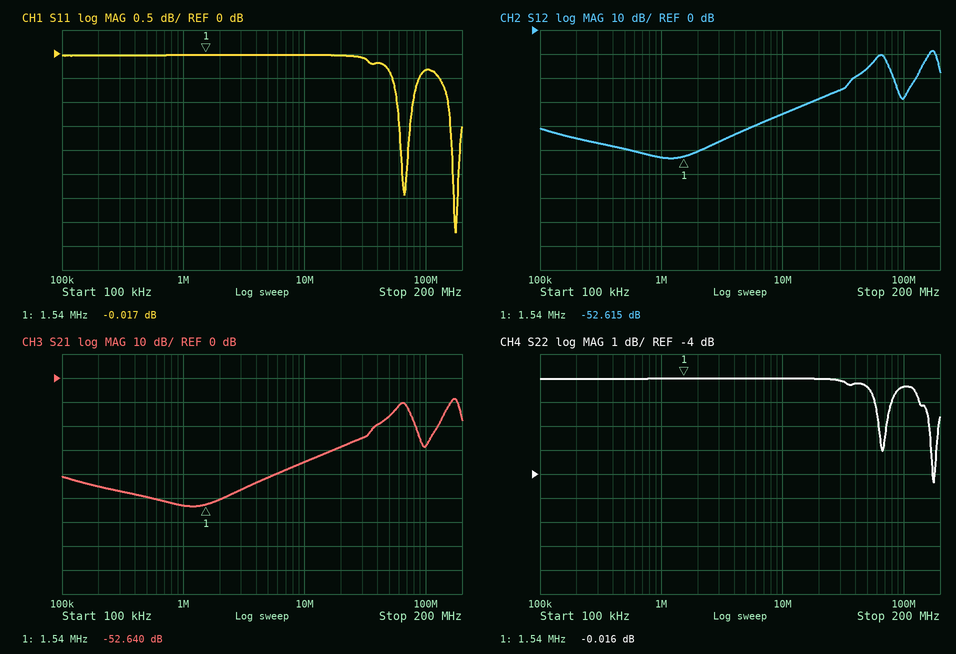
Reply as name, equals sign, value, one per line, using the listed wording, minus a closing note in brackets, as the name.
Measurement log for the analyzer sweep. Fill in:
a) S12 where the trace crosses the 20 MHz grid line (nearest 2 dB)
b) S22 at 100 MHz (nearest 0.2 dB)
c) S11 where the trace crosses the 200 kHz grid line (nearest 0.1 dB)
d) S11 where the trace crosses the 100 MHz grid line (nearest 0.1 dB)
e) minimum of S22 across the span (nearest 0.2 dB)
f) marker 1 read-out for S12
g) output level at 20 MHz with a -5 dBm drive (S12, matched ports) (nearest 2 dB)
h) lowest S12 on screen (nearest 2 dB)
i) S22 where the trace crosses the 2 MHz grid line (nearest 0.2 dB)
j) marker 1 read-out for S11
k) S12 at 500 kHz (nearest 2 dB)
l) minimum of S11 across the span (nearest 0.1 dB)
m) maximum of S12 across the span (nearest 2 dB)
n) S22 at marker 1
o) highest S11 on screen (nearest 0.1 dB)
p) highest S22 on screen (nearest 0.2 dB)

S12 where the trace crosses the 20 MHz grid line = -28 dB
S22 at 100 MHz = -0.4 dB
S11 where the trace crosses the 200 kHz grid line = 0.0 dB
S11 where the trace crosses the 100 MHz grid line = -0.3 dB
minimum of S22 across the span = -4.4 dB
marker 1 read-out for S12 = -52.615 dB
output level at 20 MHz with a -5 dBm drive (S12, matched ports) = -34 dBm
lowest S12 on screen = -54 dB
S22 where the trace crosses the 2 MHz grid line = 0.0 dB
marker 1 read-out for S11 = -0.017 dB
S12 at 500 kHz = -50 dB
minimum of S11 across the span = -3.7 dB
maximum of S12 across the span = -8 dB
S22 at marker 1 = -0.016 dB
highest S11 on screen = 0.0 dB
highest S22 on screen = 0.0 dB
